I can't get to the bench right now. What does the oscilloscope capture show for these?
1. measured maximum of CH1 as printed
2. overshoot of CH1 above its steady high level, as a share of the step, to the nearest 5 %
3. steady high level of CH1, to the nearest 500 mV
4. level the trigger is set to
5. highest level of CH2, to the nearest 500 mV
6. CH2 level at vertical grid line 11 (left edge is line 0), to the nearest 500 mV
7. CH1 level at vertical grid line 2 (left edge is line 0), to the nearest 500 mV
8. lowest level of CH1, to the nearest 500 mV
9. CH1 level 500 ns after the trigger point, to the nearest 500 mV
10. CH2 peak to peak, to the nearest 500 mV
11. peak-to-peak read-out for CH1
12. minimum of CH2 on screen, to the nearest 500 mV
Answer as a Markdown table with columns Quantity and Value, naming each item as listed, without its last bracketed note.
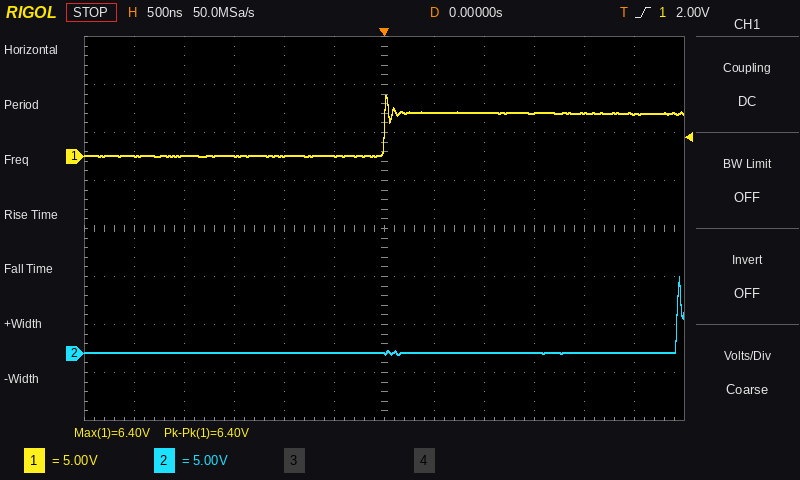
| Quantity | Value |
|---|---|
| measured maximum of CH1 as printed | 6.40 V |
| overshoot of CH1 above its steady high level, as a share of the step, to the nearest 5 % | 40 % |
| steady high level of CH1, to the nearest 500 mV | 4.5 V |
| level the trigger is set to | 2.00 V |
| highest level of CH2, to the nearest 500 mV | 8.0 V |
| CH2 level at vertical grid line 11 (left edge is line 0), to the nearest 500 mV | 0.0 V |
| CH1 level at vertical grid line 2 (left edge is line 0), to the nearest 500 mV | 0.0 V |
| lowest level of CH1, to the nearest 500 mV | 0.0 V |
| CH1 level 500 ns after the trigger point, to the nearest 500 mV | 4.5 V |
| CH2 peak to peak, to the nearest 500 mV | 8.0 V |
| peak-to-peak read-out for CH1 | 6.40 V |
| minimum of CH2 on screen, to the nearest 500 mV | 0.0 V |
